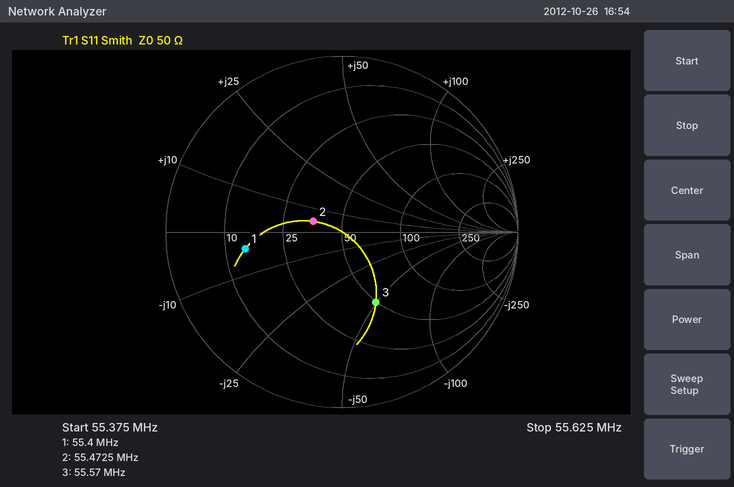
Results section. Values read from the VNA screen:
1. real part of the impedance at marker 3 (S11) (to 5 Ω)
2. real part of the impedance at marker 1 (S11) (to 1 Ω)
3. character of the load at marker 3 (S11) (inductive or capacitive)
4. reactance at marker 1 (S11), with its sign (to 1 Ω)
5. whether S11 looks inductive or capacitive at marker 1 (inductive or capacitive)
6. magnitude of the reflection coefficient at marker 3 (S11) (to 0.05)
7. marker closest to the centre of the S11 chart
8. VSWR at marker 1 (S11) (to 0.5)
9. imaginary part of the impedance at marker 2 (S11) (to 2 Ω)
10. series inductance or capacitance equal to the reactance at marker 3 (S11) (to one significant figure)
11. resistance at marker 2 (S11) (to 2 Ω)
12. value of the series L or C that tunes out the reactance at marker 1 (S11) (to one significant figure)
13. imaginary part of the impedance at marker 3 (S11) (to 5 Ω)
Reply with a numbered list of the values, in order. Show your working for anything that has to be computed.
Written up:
1. 50 Ω
2. 14 Ω
3. capacitive
4. -4 Ω
5. capacitive
6. 0.45
7. marker 2
8. 3.5
9. +4 Ω
10. C = 1/(2π × 55.57 MHz × 50 Ω) ≈ 57.3 pF, so 60 pF to one significant figure
11. 36 Ω
12. L = 4 Ω/(2π × 55.4 MHz) ≈ 11.5 nH, so 10 nH to one significant figure
13. -50 Ω
